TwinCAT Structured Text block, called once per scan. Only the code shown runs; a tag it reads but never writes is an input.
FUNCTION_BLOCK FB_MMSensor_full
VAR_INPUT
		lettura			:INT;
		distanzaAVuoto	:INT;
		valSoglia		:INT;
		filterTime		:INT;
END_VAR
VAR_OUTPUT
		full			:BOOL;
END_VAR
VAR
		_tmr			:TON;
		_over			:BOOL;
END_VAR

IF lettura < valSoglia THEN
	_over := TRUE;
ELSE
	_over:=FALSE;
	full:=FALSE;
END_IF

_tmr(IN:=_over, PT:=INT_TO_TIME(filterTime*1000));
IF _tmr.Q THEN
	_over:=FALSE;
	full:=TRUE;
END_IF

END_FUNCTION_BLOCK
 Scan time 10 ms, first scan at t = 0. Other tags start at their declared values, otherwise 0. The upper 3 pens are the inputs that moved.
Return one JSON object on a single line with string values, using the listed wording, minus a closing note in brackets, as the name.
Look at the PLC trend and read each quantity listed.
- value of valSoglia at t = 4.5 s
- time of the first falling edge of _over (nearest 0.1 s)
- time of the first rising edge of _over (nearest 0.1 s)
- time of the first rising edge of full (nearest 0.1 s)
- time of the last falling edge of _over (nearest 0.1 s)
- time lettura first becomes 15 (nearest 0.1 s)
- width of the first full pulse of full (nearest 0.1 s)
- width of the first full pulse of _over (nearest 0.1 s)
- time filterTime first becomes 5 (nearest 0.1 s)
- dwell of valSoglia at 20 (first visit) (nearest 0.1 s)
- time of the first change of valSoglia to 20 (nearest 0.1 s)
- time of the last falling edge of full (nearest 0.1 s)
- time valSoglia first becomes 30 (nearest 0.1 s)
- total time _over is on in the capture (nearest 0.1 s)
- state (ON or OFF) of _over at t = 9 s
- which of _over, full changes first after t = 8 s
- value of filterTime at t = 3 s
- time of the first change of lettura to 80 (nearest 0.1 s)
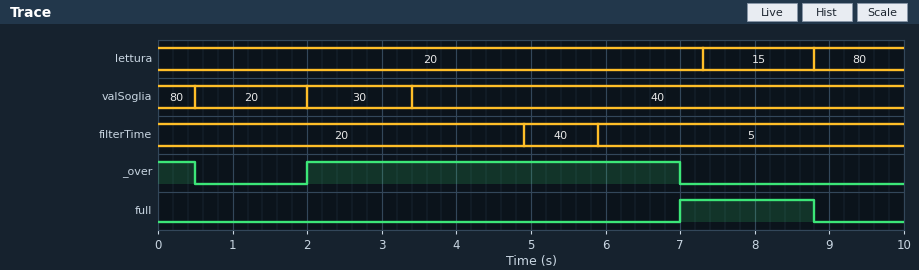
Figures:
{"value of valSoglia at t = 4.5 s": "40", "time of the first falling edge of _over": "0.5 s", "time of the first rising edge of _over": "2.0 s", "time of the first rising edge of full": "7.0 s", "time of the last falling edge of _over": "7.0 s", "time lettura first becomes 15": "7.3 s", "width of the first full pulse of full": "1.8 s", "width of the first full pulse of _over": "5.0 s", "time filterTime first becomes 5": "5.9 s", "dwell of valSoglia at 20 (first visit)": "1.5 s", "time of the first change of valSoglia to 20": "0.5 s", "time of the last falling edge of full": "8.8 s", "time valSoglia first becomes 30": "2.0 s", "total time _over is on in the capture": "5.5 s", "state (ON or OFF) of _over at t = 9 s": "OFF", "which of _over, full changes first after t = 8 s": "full", "value of filterTime at t = 3 s": "20", "time of the first change of lettura to 80": "8.8 s"}
